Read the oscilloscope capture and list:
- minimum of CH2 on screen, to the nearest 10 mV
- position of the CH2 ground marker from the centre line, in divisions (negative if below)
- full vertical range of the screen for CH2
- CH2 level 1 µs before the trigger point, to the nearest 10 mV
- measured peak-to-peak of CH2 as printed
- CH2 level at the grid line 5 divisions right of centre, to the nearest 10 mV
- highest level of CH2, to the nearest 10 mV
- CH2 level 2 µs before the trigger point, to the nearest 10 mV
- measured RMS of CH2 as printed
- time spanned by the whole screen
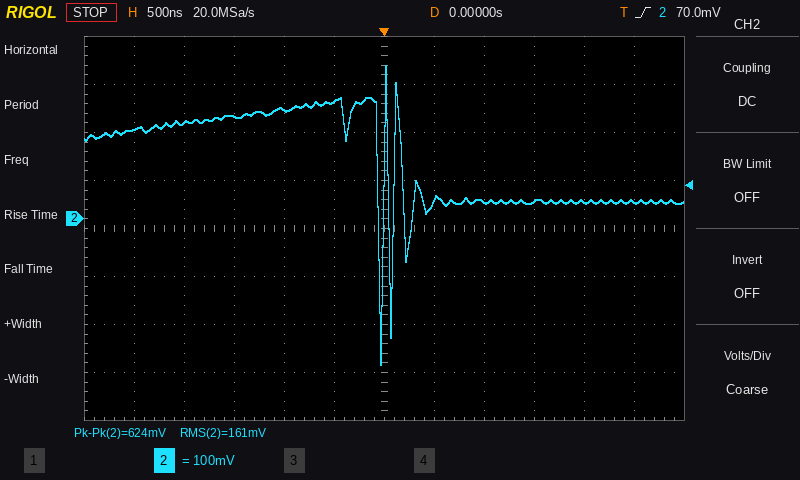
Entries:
-300 mV
+0.2 div
800 mV
230 mV
624 mV
40 mV
320 mV
200 mV
161 mV
6 µs
